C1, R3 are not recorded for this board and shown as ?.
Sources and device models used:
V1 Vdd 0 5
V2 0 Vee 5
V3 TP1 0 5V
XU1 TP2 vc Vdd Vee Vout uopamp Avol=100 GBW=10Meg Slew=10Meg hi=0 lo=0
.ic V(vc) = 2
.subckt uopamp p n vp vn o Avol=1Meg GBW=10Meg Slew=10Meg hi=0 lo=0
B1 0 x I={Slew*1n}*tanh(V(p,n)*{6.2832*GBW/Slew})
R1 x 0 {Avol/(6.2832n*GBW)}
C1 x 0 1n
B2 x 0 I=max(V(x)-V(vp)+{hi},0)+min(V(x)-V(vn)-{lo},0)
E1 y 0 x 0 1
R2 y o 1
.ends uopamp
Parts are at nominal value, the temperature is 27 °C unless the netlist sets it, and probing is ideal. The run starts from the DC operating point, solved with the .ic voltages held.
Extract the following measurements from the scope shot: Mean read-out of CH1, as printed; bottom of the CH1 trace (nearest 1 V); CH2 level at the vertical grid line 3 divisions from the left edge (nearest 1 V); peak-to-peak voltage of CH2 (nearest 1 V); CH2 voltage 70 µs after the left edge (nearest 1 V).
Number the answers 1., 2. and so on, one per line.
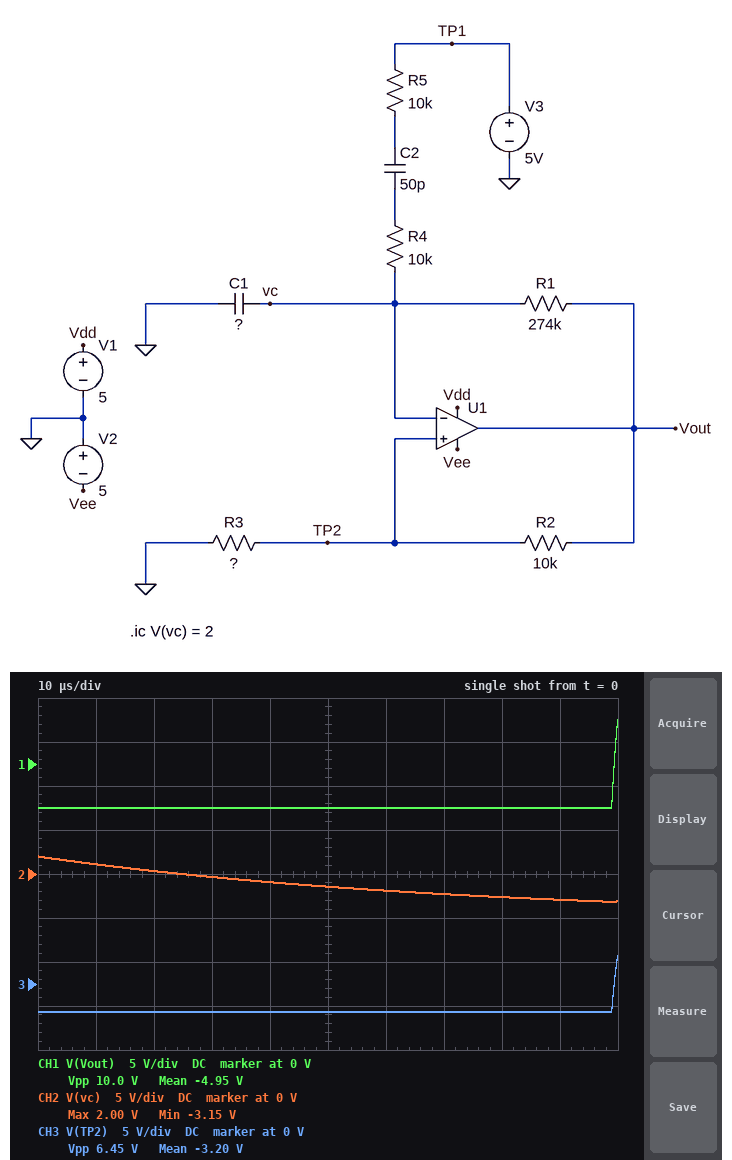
1. -4.95 V
2. -5 V
3. 0 V
4. 5 V
5. -2 V
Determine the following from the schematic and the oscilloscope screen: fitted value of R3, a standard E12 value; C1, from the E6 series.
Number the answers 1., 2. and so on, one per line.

1. 18 kΩ
2. 220 pF
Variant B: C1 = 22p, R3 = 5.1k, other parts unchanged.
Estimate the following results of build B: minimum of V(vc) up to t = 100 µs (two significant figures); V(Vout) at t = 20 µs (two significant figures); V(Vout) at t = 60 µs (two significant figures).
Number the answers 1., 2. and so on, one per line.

1. -1.7 V
2. 5.0 V
3. -5.0 V
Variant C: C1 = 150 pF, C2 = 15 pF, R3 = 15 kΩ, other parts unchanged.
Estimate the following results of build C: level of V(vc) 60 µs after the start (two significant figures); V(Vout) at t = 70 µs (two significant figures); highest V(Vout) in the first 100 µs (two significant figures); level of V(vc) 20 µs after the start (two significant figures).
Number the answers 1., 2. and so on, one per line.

1. -2.3 V
2. 5.0 V
3. 5.0 V
4. -510 mV
